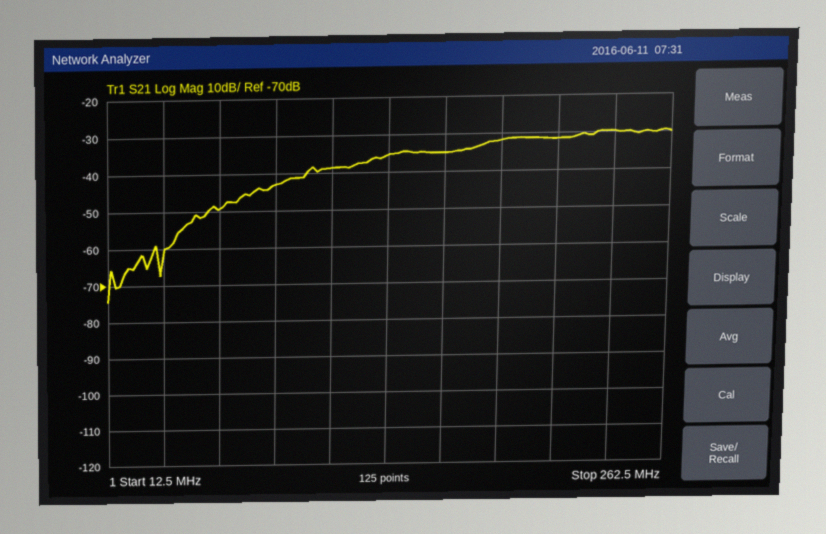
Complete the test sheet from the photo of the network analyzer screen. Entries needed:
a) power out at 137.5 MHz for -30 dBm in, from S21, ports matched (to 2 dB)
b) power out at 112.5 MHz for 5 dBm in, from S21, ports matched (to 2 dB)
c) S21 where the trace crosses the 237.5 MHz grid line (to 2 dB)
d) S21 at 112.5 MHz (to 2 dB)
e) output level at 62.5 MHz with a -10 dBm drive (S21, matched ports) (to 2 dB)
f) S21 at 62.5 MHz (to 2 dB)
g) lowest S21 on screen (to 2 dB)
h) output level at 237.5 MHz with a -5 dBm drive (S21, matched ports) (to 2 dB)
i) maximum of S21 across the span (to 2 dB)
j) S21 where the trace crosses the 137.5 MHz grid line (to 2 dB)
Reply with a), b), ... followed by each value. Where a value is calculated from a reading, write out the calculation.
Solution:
a) -30 dBm + (-36 dB) = -66 dBm
b) 5 dBm + (-38 dB) = -34 dBm
c) -30 dB
d) -38 dB
e) -10 dBm + (-50 dB) = -60 dBm
f) -50 dB
g) -74 dB
h) -5 dBm + (-30 dB) = -34 dBm
i) -30 dB
j) -36 dB
